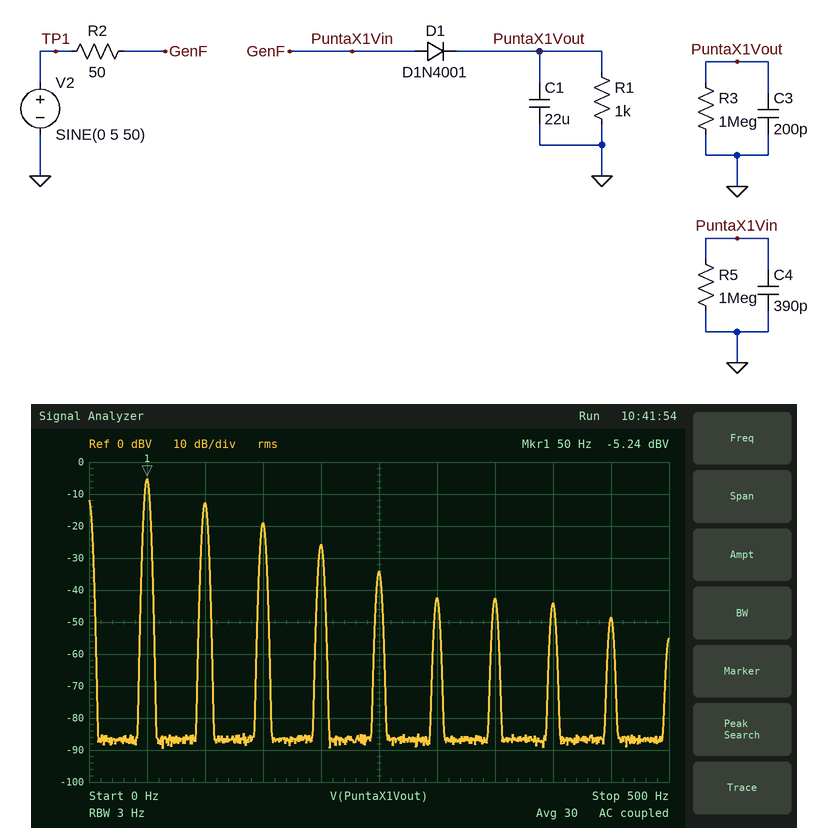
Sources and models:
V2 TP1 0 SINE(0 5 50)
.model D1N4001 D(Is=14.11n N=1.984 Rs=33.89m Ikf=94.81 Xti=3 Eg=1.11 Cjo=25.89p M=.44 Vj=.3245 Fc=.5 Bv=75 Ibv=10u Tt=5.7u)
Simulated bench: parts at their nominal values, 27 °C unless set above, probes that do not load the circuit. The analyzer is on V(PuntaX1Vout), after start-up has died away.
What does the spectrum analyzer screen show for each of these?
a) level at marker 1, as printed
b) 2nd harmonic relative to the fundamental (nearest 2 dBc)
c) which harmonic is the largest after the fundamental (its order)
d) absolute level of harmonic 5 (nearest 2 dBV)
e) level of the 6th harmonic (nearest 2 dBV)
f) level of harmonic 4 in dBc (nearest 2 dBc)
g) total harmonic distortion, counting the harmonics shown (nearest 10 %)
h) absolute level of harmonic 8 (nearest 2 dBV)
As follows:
-5.24 dBV
-8 dBc
2
-34 dBV
-42 dBV
-20 dBc
50 %
-44 dBV
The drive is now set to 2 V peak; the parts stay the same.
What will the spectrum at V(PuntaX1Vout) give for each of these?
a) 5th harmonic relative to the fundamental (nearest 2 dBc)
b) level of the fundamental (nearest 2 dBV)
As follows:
-28 dBc
-16 dBV
